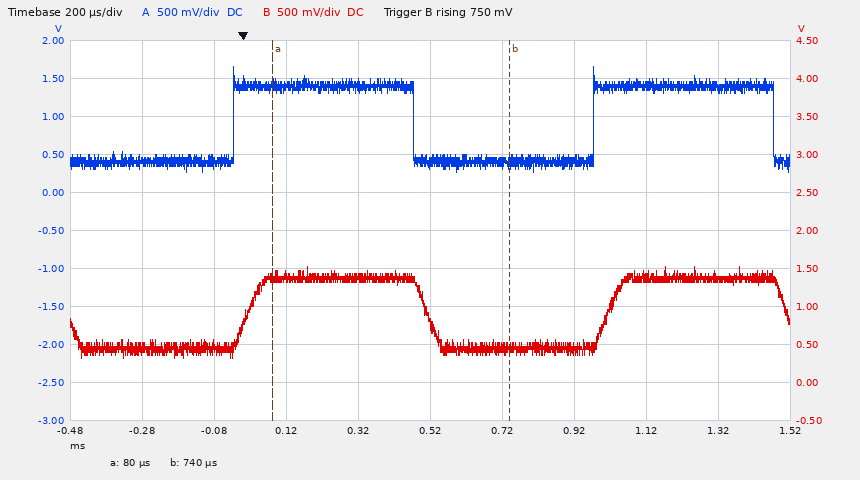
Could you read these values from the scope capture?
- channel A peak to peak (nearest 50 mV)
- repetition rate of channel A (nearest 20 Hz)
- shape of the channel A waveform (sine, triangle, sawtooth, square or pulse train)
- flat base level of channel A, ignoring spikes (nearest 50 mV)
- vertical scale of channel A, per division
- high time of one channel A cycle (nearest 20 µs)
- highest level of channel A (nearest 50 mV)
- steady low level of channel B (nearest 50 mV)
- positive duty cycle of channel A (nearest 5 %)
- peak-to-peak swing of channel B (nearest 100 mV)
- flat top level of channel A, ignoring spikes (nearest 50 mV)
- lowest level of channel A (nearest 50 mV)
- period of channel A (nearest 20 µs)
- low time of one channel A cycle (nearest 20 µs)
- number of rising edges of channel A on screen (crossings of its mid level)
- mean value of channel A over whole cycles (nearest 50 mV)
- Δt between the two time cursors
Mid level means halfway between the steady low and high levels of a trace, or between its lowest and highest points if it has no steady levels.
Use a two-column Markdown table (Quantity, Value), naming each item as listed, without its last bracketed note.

| Quantity | Value |
|---|---|
| channel A peak to peak | 1.40 V |
| repetition rate of channel A | 1.00 kHz |
| shape of the channel A waveform | square |
| flat base level of channel A, ignoring spikes | 400 mV |
| vertical scale of channel A, per division | 500 mV |
| high time of one channel A cycle | 500 µs |
| highest level of channel A | 1.65 V |
| steady low level of channel B | 450 mV |
| positive duty cycle of channel A | 50 % |
| peak-to-peak swing of channel B | 1.20 V |
| flat top level of channel A, ignoring spikes | 1.40 V |
| lowest level of channel A | 250 mV |
| period of channel A | 1.00 ms |
| low time of one channel A cycle | 500 µs |
| number of rising edges of channel A on screen | 2 |
| mean value of channel A over whole cycles | 900 mV |
| Δt between the two time cursors | 660 µs |
